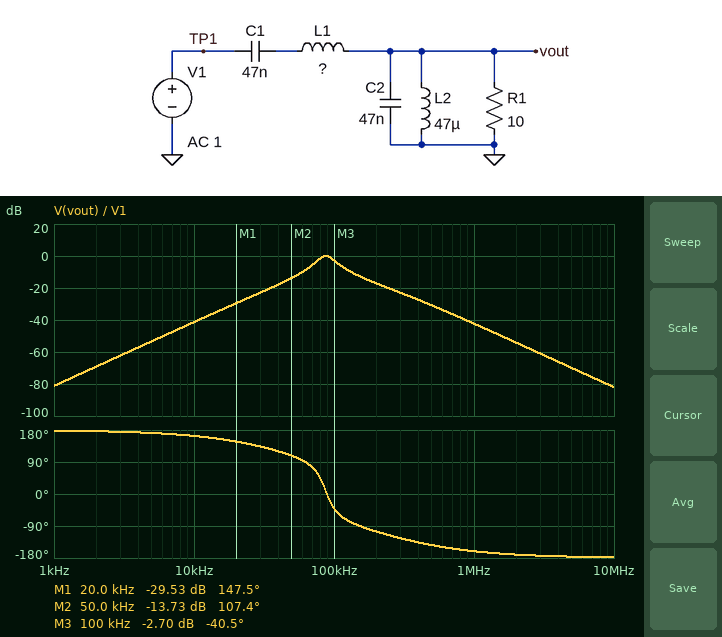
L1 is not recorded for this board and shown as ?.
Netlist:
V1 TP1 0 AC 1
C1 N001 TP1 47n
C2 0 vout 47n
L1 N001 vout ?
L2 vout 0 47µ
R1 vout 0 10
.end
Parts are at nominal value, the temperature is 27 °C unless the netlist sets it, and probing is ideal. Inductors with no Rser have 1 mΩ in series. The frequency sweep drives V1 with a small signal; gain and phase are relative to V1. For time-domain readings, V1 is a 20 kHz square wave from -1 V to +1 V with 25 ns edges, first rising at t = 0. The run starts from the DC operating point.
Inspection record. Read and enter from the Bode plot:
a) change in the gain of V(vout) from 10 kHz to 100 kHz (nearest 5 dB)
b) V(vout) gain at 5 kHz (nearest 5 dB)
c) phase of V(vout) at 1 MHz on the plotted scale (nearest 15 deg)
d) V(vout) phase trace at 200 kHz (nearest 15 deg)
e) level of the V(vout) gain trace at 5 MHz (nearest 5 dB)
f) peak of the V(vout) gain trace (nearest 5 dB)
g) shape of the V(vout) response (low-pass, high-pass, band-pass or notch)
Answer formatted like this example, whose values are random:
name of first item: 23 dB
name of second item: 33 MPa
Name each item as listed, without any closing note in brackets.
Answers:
change in the gain of V(vout) from 10 kHz to 100 kHz: 40 dB
V(vout) gain at 5 kHz: -55 dB
phase of V(vout) at 1 MHz on the plotted scale: -165 deg
V(vout) phase trace at 200 kHz: -105 deg
level of the V(vout) gain trace at 5 MHz: -70 dB
peak of the V(vout) gain trace: 0 dB
shape of the V(vout) response: band-pass
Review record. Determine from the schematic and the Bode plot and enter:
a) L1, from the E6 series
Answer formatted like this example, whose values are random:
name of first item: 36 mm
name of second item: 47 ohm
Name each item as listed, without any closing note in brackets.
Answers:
L1, from the E6 series: 68 µH
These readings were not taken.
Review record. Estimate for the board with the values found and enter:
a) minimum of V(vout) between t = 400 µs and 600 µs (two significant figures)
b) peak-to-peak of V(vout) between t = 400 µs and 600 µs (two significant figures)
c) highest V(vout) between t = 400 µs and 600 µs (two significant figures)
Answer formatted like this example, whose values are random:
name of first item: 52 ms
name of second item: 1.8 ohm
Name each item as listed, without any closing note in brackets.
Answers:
minimum of V(vout) between t = 400 µs and 600 µs: -340 mV
peak-to-peak of V(vout) between t = 400 µs and 600 µs: 690 mV
highest V(vout) between t = 400 µs and 600 µs: 340 mV
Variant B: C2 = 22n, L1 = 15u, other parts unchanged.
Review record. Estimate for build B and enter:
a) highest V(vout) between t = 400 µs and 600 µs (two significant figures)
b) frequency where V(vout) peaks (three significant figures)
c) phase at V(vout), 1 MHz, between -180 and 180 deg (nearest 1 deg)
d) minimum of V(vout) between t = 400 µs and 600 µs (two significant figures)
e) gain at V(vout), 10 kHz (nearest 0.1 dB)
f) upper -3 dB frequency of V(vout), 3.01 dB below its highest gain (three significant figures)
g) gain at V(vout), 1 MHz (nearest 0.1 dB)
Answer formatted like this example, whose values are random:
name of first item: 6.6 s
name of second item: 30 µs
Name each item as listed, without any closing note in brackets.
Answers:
highest V(vout) between t = 400 µs and 600 µs: 720 mV
frequency where V(vout) peaks: 195 kHz
phase at V(vout), 1 MHz, between -180 and 180 deg: -141 deg
minimum of V(vout) between t = 400 µs and 600 µs: -720 mV
gain at V(vout), 10 kHz: -41.4 dB
upper -3 dB frequency of V(vout), 3.01 dB below its highest gain: 265 kHz
gain at V(vout), 1 MHz: -23.2 dB
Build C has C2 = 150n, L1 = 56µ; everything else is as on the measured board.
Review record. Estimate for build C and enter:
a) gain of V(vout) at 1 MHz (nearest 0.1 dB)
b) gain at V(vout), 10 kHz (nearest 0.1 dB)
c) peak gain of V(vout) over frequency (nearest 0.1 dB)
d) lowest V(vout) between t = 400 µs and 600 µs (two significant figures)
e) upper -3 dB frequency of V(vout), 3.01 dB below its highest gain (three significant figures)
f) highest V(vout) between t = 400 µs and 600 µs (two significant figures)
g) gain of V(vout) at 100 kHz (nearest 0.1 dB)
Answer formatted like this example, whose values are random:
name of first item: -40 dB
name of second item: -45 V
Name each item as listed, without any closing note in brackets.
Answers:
gain of V(vout) at 1 MHz: -50.3 dB
gain at V(vout), 10 kHz: -41.2 dB
peak gain of V(vout) over frequency: 1.6 dB
lowest V(vout) between t = 400 µs and 600 µs: -450 mV
upper -3 dB frequency of V(vout), 3.01 dB below its highest gain: 116 kHz
highest V(vout) between t = 400 µs and 600 µs: 450 mV
gain of V(vout) at 100 kHz: 0.6 dB
